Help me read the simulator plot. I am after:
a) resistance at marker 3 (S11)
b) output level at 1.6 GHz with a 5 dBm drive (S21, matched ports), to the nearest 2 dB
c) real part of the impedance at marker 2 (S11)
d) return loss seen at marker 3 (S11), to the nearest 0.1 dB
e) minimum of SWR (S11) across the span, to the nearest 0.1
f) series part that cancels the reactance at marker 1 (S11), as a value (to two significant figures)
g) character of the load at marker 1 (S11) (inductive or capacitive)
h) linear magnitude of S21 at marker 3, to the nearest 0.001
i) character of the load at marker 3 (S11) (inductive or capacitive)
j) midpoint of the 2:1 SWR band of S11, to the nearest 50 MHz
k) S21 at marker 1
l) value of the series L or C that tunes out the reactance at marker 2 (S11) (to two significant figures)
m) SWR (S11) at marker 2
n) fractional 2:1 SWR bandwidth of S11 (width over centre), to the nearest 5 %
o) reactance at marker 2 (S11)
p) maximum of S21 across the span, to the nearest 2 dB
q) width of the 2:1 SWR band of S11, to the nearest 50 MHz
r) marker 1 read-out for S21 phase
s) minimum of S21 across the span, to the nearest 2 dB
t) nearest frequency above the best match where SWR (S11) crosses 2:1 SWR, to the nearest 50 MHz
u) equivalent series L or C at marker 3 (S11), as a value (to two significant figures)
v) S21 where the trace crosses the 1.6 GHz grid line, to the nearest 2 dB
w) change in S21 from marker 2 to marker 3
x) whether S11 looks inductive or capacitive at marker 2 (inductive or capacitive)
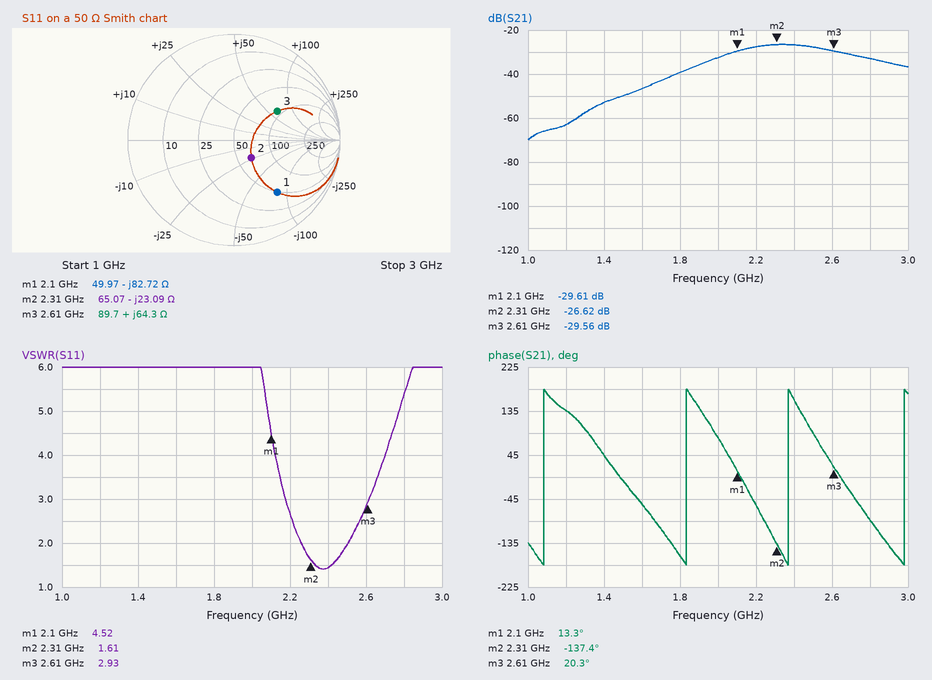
89.7 Ω
-42 dBm
65.07 Ω
6.2 dB
1.4
6.3 nH
capacitive
0.033
inductive
2.40 GHz
-29.61 dB
1.6 nH
1.61
10 %
-23.09 Ω
-26 dB
250 MHz
13.3°
-70 dB
2.50 GHz
3.9 nH
-46 dB
-2.94 dB
capacitive
